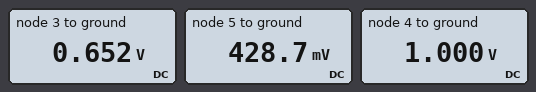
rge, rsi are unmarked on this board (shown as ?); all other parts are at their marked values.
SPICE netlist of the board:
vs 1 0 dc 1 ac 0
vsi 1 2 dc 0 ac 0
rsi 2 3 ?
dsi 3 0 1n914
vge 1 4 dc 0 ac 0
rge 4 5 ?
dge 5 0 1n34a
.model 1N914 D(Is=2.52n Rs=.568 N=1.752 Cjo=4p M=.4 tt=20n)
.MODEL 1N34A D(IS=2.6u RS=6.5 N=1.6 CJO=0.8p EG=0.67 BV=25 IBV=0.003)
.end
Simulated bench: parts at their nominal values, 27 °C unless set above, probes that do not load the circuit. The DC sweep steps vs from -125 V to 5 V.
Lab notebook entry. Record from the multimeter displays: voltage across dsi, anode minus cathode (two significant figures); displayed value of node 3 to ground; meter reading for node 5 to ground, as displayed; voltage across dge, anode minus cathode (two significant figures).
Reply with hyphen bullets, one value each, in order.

- 650 mV
- 0.652 V
- 428.7 mV
- 430 mV
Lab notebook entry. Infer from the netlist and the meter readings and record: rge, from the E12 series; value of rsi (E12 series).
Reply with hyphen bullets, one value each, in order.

- 47 Ω
- 82 Ω
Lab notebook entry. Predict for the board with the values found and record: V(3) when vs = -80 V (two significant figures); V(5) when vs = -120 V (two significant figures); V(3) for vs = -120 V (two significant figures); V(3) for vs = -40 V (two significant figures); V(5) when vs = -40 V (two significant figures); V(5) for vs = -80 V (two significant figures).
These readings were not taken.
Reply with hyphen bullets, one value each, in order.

- -80 V
- -37 V
- -120 V
- -40 V
- -27 V
- -32 V
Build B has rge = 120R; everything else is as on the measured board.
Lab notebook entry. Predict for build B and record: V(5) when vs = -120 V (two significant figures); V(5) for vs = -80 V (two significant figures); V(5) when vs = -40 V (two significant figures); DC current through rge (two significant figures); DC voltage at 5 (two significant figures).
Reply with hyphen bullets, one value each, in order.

- -30 V
- -28 V
- -26 V
- 5.4 mA
- 350 mV
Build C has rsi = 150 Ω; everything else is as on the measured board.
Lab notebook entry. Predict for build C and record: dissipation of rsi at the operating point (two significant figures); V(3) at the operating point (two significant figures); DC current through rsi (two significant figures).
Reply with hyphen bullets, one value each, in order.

- 930 µW
- 630 mV
- 2.5 mA
